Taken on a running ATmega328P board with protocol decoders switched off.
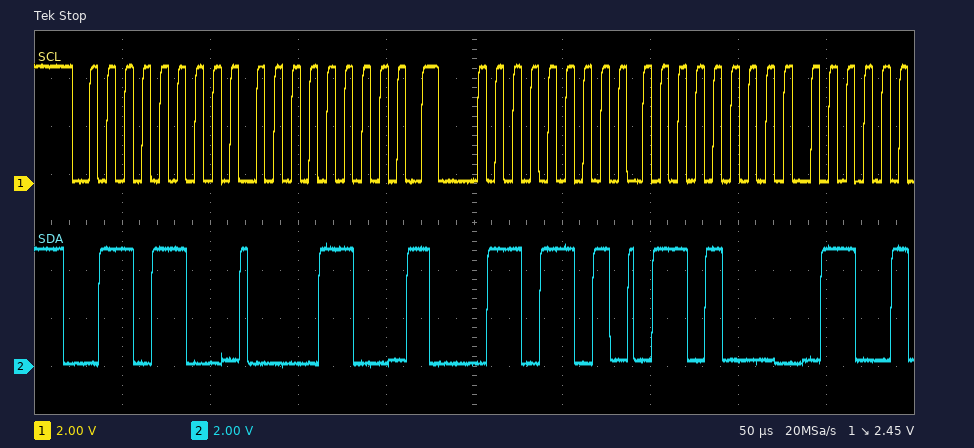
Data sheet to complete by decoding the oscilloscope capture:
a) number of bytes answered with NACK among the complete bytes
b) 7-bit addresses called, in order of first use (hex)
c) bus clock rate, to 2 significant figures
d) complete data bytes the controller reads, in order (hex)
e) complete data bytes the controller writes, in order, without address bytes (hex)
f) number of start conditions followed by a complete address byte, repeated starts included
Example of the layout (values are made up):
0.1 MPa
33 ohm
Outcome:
0
0x36
100 kHz
68
0C
2
